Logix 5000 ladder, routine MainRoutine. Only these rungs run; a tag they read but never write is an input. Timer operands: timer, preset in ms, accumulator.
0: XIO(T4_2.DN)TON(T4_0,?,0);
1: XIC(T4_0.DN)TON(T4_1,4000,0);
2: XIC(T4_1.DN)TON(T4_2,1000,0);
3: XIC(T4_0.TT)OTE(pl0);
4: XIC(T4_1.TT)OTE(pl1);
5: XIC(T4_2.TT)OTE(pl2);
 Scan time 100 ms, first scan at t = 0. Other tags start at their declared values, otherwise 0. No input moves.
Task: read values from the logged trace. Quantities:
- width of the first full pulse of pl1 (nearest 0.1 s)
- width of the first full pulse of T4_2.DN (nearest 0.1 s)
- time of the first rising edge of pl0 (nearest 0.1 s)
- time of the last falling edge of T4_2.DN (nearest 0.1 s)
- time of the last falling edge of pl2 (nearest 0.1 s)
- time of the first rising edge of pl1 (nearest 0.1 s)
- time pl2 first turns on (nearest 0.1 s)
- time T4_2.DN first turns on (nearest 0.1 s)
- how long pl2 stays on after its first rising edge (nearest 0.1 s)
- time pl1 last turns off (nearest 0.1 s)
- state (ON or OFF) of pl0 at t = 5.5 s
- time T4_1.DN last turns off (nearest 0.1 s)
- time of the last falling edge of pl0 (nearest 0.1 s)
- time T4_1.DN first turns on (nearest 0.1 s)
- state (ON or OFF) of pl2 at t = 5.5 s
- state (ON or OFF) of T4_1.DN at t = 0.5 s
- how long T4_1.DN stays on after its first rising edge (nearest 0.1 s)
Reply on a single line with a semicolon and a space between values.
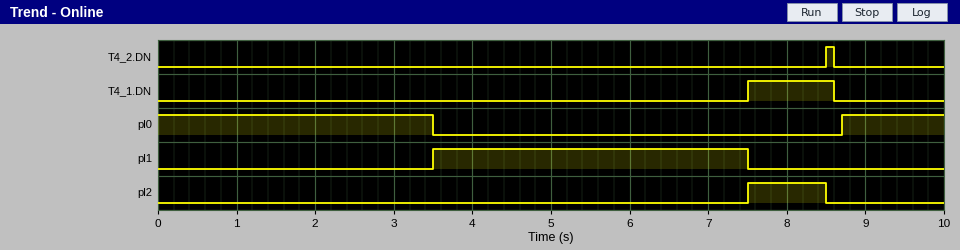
4.0 s; 0.1 s; 8.7 s; 8.6 s; 8.5 s; 3.5 s; 7.5 s; 8.5 s; 1.0 s; 7.5 s; OFF; 8.6 s; 3.5 s; 7.5 s; OFF; OFF; 1.1 s
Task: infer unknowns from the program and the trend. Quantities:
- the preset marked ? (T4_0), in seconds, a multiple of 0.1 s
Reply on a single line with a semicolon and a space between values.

3.5 s
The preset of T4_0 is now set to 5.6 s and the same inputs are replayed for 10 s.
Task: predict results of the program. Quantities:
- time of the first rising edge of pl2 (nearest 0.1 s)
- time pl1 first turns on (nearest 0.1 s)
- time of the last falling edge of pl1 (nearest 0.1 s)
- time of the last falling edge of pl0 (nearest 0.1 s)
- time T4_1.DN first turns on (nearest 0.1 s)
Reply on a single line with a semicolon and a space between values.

9.6 s; 5.6 s; 9.6 s; 5.6 s; 9.6 s
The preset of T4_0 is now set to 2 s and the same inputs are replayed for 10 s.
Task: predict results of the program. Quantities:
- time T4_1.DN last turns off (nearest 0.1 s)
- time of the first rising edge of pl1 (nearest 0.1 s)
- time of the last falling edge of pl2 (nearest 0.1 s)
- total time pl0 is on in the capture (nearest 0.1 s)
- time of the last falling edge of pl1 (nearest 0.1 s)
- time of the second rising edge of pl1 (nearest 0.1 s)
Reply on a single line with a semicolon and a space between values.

7.1 s; 2.0 s; 7.0 s; 4.0 s; 6.0 s; 9.2 s
